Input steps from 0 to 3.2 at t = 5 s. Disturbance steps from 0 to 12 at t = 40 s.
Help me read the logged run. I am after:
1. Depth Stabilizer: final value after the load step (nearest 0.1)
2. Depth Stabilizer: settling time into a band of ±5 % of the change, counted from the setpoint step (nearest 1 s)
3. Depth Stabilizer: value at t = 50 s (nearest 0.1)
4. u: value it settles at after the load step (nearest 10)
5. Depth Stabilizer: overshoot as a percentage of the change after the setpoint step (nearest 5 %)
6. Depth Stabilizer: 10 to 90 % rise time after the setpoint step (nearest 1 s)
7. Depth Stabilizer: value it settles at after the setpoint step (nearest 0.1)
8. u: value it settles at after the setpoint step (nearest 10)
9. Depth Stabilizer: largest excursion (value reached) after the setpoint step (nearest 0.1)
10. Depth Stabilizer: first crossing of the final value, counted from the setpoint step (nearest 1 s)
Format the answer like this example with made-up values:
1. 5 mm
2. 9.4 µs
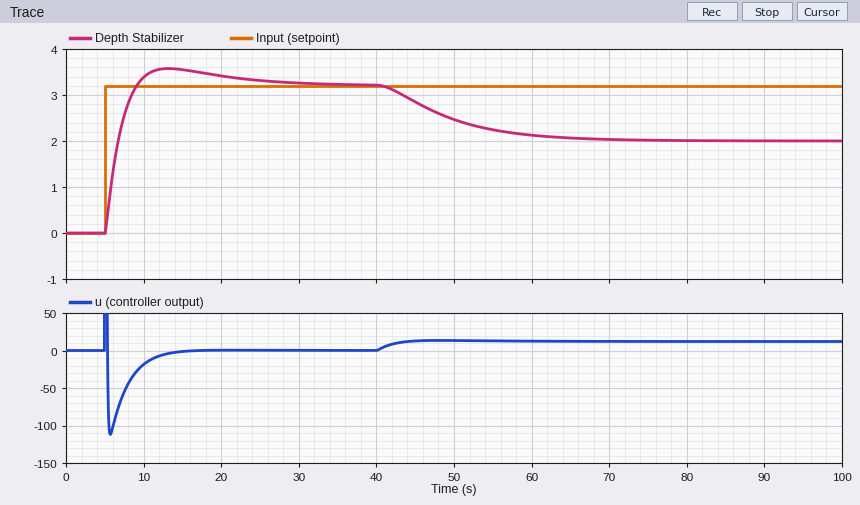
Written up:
1. 2.0
2. 17 s
3. 2.5
4. 10
5. 10 %
6. 3 s
7. 3.2
8. 0
9. 3.6
10. 4 s
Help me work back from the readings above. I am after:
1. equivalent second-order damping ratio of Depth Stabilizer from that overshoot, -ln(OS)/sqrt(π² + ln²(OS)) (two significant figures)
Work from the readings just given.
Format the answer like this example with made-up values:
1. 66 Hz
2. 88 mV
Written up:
1. 0.59
